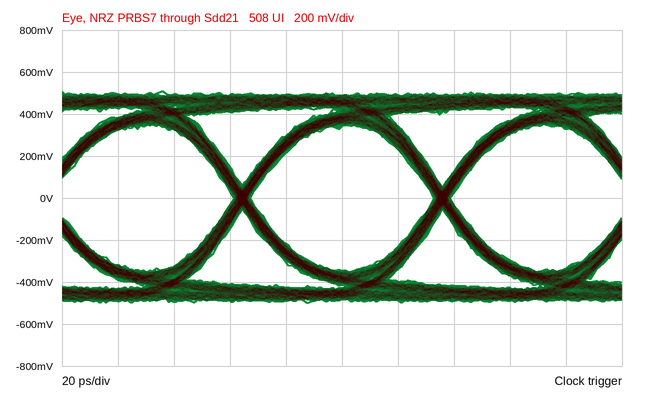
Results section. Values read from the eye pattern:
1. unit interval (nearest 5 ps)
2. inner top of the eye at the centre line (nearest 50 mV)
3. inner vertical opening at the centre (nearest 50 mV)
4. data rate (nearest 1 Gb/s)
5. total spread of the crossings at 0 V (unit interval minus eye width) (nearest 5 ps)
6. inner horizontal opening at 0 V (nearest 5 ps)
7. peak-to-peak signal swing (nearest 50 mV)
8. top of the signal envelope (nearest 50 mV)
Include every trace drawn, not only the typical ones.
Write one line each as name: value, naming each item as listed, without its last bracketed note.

unit interval: 70 ps
inner top of the eye at the centre line: 350 mV
inner vertical opening at the centre: 700 mV
data rate: 14 Gb/s
total spread of the crossings at 0 V (unit interval minus eye width): 5 ps
inner horizontal opening at 0 V: 65 ps
peak-to-peak signal swing: 1.00 V
top of the signal envelope: 500 mV
